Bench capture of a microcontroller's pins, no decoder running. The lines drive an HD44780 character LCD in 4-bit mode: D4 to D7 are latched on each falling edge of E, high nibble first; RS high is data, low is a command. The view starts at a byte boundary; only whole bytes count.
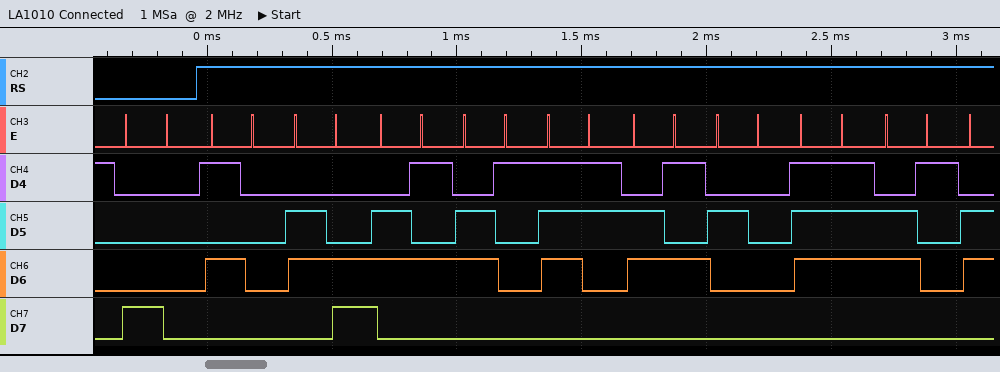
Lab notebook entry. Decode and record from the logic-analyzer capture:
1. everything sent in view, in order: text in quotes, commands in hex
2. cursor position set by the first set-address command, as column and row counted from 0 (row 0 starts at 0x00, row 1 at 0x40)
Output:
0x80 "Please wa"
column 0, row 0
